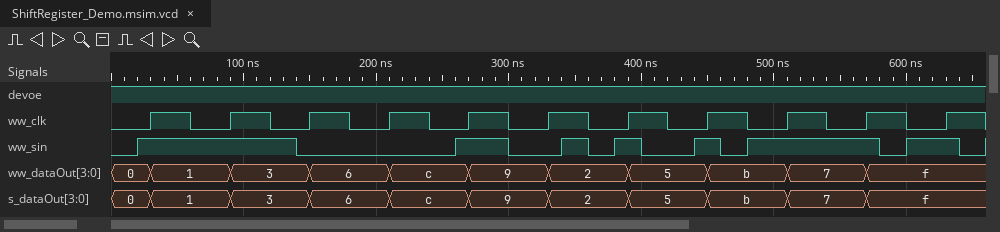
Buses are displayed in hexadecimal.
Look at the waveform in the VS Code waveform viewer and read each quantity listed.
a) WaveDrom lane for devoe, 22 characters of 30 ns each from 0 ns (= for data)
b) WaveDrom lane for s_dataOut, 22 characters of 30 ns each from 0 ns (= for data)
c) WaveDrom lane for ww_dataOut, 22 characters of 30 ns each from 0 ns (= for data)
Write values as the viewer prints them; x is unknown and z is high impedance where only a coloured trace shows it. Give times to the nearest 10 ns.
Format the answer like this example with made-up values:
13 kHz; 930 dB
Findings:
{name: 'devoe', wave: '1.....................'}; {name: 's_dataOut', wave: '==.=.=.=.=.=.=.=.=.=..', data: '0 1 3 6 c 9 2 5 b 7 f'}; {name: 'ww_dataOut', wave: '==.=.=.=.=.=.=.=.=.=..', data: '0 1 3 6 c 9 2 5 b 7 f'}
